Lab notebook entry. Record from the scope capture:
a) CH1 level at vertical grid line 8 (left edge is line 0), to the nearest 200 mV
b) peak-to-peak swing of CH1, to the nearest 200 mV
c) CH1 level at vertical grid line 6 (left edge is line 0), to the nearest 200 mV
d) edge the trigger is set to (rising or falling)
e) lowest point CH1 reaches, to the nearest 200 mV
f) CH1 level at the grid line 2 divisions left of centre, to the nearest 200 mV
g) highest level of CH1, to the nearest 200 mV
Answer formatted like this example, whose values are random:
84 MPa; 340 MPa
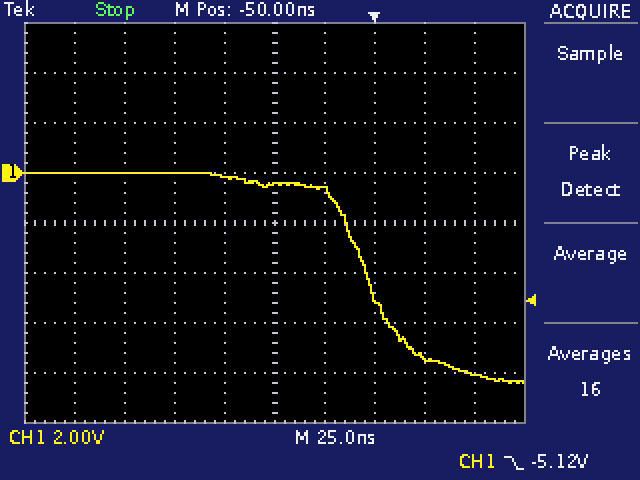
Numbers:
-7.4 V; 8.4 V; -600 mV; falling; -8.4 V; 0.0 V; 0.0 V
